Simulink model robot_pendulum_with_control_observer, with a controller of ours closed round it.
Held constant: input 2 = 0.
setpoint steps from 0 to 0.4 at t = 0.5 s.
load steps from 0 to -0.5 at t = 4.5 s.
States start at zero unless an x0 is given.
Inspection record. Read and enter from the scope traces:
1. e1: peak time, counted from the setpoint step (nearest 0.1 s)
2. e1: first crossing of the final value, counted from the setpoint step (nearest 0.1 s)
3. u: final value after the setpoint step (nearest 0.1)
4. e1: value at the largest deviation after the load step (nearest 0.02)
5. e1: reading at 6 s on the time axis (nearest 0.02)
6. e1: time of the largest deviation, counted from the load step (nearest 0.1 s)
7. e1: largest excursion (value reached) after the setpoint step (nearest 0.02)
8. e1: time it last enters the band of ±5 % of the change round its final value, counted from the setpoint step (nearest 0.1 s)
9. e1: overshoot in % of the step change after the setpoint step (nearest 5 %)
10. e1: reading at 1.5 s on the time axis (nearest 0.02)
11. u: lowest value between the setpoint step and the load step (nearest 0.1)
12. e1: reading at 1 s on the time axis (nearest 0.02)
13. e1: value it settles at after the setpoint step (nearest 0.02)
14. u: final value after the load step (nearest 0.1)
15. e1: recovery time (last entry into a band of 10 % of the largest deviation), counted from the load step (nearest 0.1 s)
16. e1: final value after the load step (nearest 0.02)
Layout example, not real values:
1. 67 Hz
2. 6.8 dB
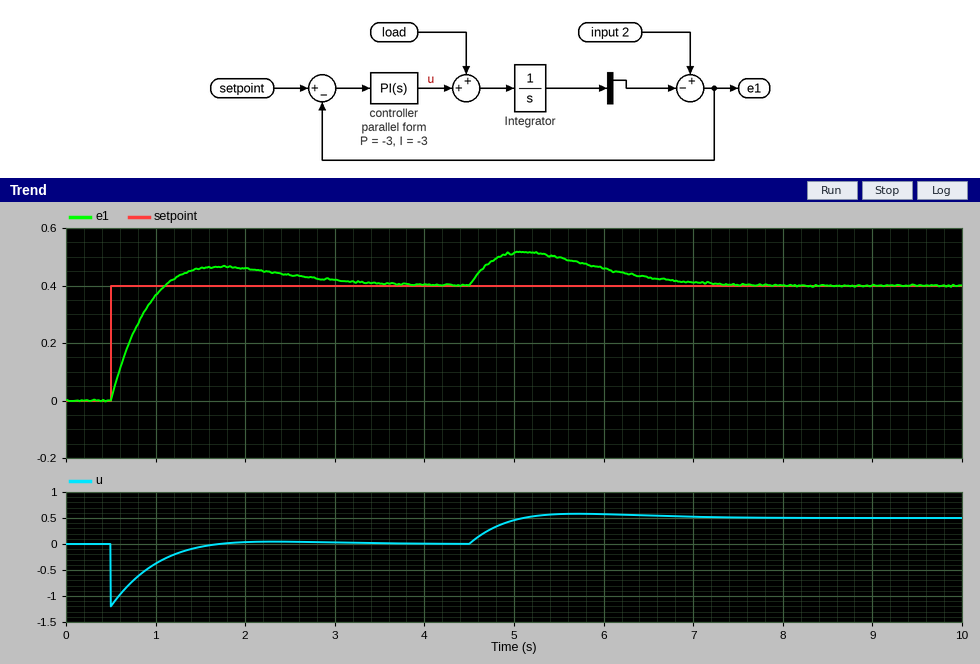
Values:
1. 1.2 s
2. 0.6 s
3. 0.0
4. 0.52
5. 0.46
6. 0.6 s
7. 0.46
8. 2.5 s
9. 15 %
10. 0.46
11. -1.2
12. 0.36
13. 0.40
14. 0.5
15. 2.5 s
16. 0.40
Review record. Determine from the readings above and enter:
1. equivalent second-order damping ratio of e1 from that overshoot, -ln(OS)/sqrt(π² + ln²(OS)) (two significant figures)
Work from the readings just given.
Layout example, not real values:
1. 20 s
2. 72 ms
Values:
1. 0.52
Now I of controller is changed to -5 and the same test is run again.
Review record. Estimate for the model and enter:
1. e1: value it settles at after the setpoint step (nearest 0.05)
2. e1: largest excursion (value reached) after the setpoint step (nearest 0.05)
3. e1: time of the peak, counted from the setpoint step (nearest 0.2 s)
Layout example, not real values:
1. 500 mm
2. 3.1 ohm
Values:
1. 0.40
2. 0.50
3. 1.0 s
